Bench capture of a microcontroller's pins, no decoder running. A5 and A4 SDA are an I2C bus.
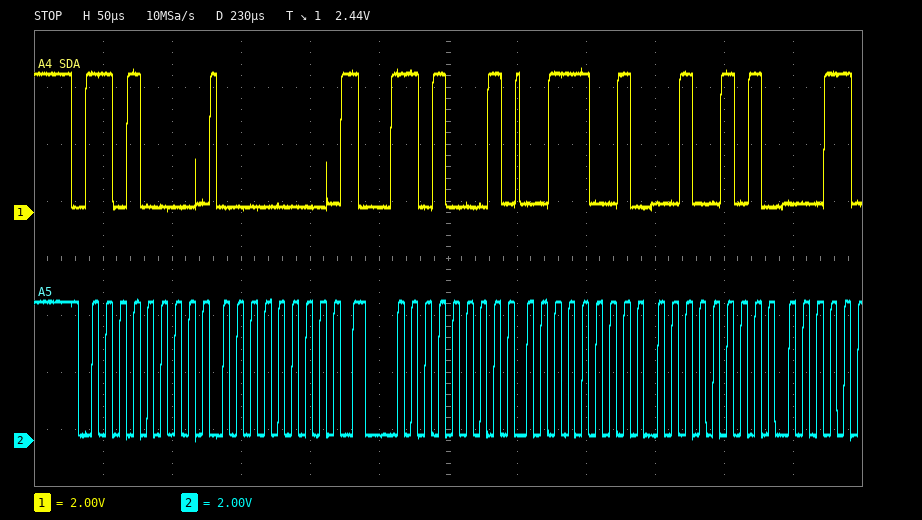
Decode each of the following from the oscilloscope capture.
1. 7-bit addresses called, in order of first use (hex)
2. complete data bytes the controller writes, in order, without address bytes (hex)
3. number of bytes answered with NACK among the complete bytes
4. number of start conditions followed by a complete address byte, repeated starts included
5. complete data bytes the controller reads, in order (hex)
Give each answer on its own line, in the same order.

0x68
00
0
2
39 25
